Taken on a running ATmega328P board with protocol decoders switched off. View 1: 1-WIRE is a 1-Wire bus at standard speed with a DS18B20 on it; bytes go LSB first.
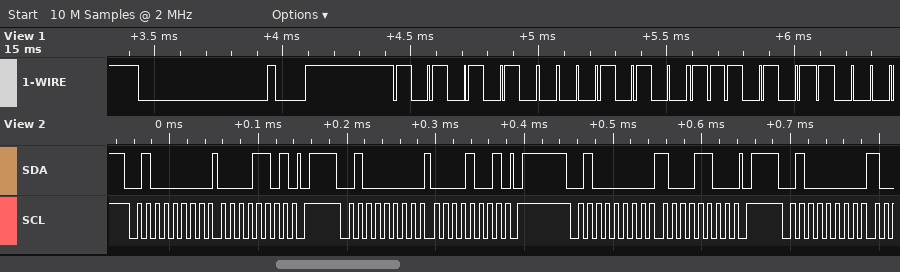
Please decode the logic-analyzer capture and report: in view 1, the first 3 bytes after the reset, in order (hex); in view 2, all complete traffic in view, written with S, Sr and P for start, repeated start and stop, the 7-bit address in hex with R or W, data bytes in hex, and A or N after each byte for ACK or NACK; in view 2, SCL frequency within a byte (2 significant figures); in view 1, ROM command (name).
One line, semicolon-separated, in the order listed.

55 28 D7; S 20W A 0D A P S 20W A 09 A P S 20W A 8C A P S 20W A; 100 kHz; Match ROM
